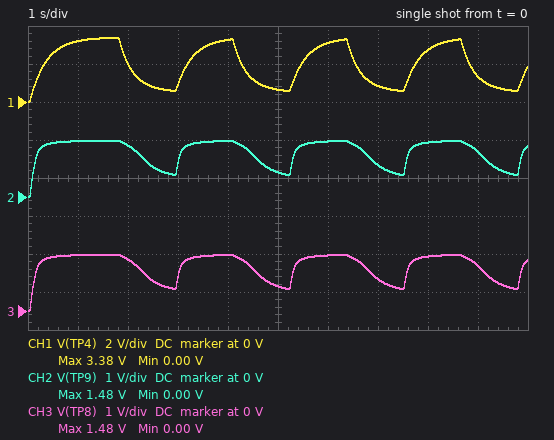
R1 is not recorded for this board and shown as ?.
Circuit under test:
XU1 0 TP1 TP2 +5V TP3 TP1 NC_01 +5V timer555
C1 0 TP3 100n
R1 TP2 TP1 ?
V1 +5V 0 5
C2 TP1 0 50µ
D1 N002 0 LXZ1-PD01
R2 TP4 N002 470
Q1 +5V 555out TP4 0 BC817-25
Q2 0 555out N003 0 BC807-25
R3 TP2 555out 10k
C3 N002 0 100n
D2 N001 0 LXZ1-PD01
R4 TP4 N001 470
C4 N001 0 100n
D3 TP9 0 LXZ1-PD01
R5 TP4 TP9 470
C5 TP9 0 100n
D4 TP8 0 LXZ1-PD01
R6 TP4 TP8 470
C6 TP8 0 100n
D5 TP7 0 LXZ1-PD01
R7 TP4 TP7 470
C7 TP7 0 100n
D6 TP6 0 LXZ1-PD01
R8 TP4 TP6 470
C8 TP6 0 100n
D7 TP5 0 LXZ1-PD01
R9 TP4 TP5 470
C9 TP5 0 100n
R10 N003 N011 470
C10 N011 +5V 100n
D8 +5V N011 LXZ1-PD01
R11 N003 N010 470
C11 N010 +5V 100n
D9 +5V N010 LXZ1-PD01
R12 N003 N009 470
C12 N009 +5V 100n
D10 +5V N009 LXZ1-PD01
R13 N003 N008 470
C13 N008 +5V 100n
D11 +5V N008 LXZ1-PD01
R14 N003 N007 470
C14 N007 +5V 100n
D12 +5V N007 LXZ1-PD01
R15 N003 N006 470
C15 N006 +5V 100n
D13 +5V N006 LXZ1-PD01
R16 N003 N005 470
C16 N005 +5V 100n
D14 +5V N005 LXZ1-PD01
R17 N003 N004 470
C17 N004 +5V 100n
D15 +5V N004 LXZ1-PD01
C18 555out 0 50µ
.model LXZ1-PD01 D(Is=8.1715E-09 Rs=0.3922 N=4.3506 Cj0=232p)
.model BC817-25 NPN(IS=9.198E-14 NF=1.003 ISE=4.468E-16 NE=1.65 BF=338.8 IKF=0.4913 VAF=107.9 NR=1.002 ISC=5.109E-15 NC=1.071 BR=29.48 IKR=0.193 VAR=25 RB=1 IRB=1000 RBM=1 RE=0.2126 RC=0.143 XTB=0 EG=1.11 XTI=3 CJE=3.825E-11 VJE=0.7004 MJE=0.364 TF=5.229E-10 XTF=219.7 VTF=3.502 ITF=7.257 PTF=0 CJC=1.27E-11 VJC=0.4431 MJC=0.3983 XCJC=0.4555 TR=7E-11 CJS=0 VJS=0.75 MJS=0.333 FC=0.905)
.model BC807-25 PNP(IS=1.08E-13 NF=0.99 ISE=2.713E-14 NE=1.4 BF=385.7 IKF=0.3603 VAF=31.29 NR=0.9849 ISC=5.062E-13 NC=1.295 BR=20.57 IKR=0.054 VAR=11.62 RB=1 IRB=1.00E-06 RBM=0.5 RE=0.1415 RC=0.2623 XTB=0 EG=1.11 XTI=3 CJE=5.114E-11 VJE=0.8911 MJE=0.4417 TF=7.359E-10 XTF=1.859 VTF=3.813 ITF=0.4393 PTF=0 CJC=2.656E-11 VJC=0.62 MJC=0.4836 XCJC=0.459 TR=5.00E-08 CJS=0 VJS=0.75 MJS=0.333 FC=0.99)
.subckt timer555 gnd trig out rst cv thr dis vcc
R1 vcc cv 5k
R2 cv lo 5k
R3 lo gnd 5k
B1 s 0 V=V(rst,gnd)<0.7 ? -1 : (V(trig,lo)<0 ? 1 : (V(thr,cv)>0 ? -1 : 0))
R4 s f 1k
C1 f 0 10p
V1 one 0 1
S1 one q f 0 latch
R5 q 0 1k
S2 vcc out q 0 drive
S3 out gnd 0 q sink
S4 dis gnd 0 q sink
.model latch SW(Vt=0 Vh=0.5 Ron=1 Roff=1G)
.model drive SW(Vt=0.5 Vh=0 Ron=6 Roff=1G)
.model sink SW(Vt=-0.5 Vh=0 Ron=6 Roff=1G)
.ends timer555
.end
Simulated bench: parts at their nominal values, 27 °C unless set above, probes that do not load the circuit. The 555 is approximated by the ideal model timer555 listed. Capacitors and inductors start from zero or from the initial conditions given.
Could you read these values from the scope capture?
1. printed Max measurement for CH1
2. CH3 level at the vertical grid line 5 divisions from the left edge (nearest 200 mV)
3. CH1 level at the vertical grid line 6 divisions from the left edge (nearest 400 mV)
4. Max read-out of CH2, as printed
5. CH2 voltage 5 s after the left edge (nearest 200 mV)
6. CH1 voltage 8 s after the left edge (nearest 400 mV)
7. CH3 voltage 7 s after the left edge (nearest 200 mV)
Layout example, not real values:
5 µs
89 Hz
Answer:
3.38 V
600 mV
3.2 V
1.48 V
600 mV
2.8 V
800 mV
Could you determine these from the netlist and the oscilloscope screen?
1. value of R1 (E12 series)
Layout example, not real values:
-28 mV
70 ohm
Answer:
33 kΩ
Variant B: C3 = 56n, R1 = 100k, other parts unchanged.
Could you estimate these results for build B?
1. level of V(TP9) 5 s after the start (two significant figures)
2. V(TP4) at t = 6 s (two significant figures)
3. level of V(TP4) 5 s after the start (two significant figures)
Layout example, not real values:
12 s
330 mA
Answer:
1.5 V
1.0 V
3.4 V
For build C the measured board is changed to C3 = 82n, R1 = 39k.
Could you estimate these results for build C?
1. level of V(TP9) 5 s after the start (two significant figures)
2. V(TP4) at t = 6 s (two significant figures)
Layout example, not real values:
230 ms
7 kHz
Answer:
1.4 V
570 mV
